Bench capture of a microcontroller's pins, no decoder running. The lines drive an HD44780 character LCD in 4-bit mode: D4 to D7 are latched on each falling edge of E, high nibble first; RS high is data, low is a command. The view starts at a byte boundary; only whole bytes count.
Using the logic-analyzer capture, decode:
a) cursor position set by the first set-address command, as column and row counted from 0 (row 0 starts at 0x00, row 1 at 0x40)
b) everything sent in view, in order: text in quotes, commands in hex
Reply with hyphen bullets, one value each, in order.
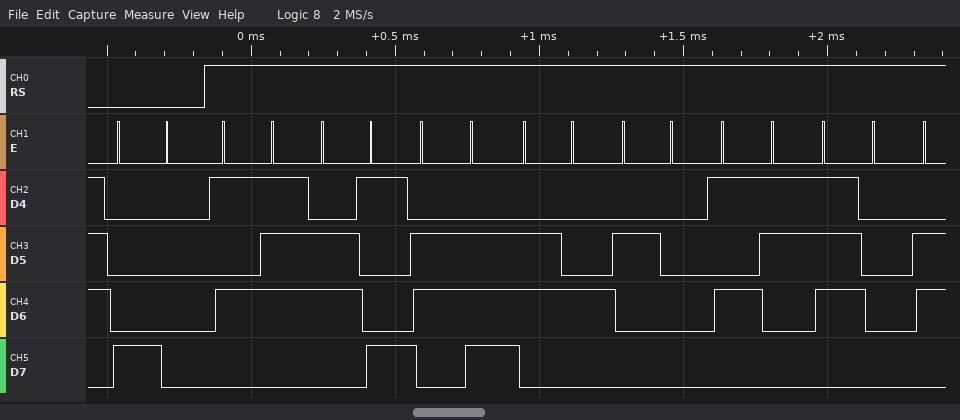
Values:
- column 0, row 0
- 0x80 "Wind Sp"
